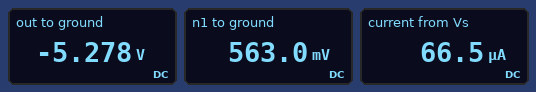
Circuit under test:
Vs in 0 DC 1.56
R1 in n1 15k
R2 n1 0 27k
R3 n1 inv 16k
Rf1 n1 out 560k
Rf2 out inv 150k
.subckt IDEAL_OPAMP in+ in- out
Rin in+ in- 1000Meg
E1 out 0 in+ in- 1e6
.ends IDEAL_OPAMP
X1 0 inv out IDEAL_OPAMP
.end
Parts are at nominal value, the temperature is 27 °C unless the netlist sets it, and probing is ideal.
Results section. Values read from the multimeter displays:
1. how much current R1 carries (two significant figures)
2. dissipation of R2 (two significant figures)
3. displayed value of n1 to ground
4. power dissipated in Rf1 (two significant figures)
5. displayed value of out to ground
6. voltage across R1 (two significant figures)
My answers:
66 µA
12 µW
563.0 mV
61 µW
-5.278 V
1.0 V
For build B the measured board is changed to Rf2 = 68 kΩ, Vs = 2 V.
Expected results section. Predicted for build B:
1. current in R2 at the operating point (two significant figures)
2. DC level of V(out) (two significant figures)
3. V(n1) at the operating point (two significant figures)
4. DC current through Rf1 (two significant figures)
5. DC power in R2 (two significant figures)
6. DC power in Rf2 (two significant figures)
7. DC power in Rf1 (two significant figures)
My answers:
28 µA
-3.2 V
760 mV
7.1 µA
21 µW
150 µW
28 µW
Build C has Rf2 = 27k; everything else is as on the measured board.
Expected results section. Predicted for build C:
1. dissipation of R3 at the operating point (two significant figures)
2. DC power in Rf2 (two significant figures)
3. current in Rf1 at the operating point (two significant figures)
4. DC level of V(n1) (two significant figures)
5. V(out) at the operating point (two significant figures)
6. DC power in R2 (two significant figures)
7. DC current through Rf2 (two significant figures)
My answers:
23 µW
39 µW
2.9 µA
610 mV
-1.0 V
14 µW
38 µA
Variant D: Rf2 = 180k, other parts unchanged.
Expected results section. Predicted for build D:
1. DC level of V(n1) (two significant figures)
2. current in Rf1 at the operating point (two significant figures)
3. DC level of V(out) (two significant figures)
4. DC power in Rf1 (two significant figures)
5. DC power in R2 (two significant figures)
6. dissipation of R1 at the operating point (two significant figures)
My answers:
550 mV
12 µA
-6.2 V
82 µW
11 µW
68 µW
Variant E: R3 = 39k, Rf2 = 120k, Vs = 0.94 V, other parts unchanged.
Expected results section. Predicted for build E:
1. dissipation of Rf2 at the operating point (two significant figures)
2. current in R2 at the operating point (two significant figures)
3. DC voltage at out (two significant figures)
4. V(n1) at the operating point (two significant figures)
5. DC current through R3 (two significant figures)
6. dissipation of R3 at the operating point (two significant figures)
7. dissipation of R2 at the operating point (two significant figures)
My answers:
17 µW
17 µA
-1.4 V
460 mV
12 µA
5.4 µW
7.8 µW
